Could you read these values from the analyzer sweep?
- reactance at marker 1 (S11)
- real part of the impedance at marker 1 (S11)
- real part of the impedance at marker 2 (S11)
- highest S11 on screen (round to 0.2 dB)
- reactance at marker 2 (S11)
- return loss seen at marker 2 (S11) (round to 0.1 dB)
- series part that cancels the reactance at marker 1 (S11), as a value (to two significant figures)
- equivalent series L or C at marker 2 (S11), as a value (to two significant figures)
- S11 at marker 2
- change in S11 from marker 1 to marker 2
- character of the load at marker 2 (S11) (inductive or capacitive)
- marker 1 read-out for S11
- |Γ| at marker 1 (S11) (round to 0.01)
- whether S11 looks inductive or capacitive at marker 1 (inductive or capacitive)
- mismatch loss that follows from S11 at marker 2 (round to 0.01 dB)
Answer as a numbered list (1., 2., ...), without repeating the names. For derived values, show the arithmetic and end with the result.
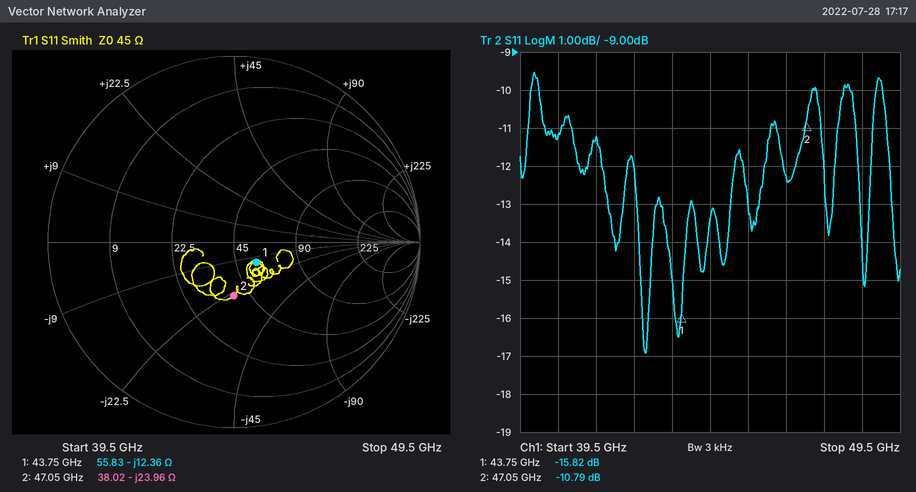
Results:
1. -12.36 Ω
2. 55.83 Ω
3. 38.02 Ω
4. -9.6 dB
5. -23.96 Ω
6. 10.8 dB
7. L = 12.36 Ω/(2π × 43.75 GHz) ≈ 45 pH
8. C = 1/(2π × 47.05 GHz × 23.96 Ω) ≈ 141 fF, so 140 fF to two significant figures
9. -10.79 dB
10. -10.79 − (-15.82) = 5.03 dB
11. capacitive
12. -15.82 dB
13. 0.16
14. capacitive
15. −10 log10(1 − 10^(-10.79/10)) ≈ 0.38 dB
